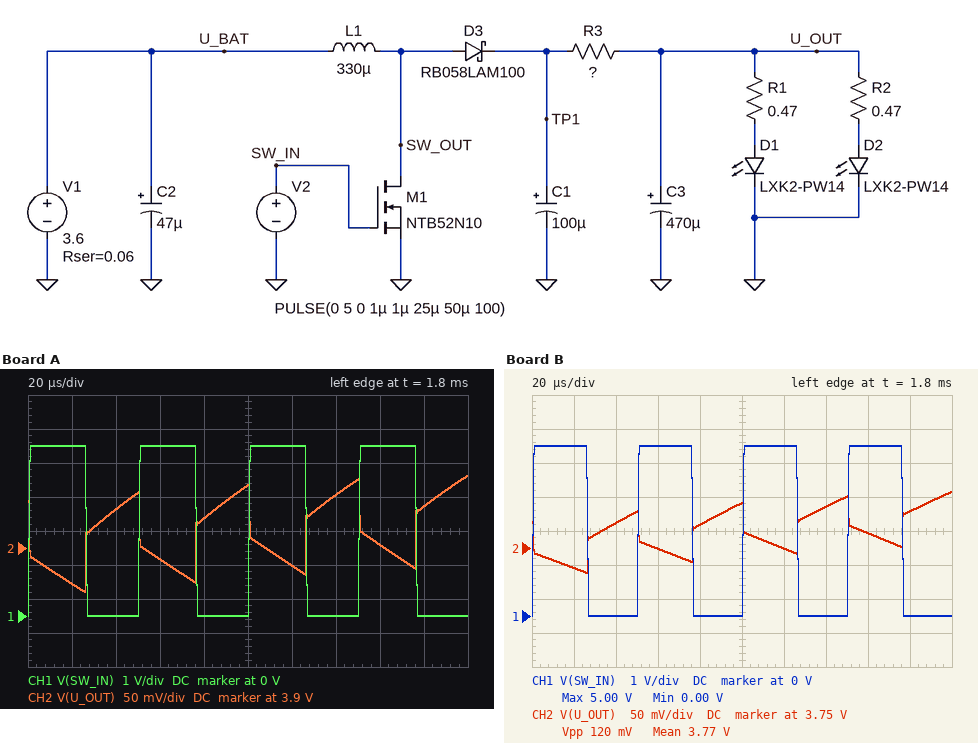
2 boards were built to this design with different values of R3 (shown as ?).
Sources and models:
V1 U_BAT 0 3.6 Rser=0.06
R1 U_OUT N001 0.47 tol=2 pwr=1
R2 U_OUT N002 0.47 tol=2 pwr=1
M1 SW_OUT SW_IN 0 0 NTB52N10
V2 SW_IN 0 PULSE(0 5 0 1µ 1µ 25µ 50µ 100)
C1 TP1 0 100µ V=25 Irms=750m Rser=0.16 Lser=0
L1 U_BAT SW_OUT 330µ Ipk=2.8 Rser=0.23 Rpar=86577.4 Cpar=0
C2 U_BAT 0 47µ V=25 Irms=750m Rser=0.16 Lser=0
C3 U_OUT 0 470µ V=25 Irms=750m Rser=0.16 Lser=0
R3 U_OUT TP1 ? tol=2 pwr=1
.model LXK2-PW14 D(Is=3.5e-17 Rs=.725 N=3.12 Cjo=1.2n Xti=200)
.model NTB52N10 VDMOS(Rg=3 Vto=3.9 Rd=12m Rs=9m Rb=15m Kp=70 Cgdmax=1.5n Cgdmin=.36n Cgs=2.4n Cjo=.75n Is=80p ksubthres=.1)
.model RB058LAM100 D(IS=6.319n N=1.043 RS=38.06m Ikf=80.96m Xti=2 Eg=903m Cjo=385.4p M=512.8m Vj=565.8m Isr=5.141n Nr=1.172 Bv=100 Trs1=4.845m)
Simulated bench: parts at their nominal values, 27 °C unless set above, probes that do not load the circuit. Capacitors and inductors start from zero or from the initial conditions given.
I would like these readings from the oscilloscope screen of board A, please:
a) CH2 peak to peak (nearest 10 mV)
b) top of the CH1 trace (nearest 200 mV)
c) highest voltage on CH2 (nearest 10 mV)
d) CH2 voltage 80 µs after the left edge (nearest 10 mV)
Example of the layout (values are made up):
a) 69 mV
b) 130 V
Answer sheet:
a) 170 mV
b) 5.0 V
c) 4.01 V
d) 3.94 V
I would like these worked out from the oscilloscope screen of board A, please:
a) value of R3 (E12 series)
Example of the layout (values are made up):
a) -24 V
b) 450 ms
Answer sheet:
a) 0.56 Ω
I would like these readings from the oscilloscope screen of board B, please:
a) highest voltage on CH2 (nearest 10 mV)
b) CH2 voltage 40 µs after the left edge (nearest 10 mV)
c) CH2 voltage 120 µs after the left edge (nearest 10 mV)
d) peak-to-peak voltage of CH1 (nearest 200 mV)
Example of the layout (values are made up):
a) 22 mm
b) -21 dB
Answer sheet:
a) 3.83 V
b) 3.79 V
c) 3.75 V
d) 5.0 V
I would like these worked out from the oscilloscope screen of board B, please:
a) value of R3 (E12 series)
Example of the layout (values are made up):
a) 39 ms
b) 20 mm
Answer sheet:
a) 1 Ω
